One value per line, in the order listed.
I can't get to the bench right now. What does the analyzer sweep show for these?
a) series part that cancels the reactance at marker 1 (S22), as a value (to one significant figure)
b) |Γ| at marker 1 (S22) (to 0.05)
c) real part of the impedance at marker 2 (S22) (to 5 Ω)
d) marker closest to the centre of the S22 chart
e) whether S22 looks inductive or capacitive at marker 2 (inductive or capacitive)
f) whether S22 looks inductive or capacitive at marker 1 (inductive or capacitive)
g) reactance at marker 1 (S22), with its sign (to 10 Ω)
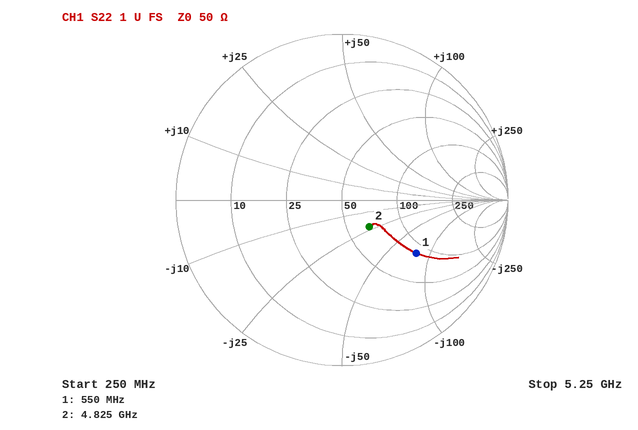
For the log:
20 nH
0.55
65 Ω
marker 2
capacitive
capacitive
-80 Ω
